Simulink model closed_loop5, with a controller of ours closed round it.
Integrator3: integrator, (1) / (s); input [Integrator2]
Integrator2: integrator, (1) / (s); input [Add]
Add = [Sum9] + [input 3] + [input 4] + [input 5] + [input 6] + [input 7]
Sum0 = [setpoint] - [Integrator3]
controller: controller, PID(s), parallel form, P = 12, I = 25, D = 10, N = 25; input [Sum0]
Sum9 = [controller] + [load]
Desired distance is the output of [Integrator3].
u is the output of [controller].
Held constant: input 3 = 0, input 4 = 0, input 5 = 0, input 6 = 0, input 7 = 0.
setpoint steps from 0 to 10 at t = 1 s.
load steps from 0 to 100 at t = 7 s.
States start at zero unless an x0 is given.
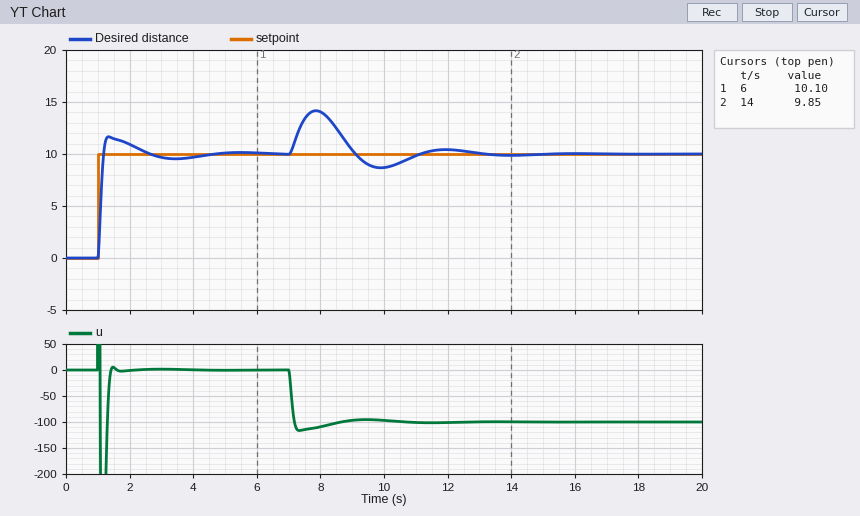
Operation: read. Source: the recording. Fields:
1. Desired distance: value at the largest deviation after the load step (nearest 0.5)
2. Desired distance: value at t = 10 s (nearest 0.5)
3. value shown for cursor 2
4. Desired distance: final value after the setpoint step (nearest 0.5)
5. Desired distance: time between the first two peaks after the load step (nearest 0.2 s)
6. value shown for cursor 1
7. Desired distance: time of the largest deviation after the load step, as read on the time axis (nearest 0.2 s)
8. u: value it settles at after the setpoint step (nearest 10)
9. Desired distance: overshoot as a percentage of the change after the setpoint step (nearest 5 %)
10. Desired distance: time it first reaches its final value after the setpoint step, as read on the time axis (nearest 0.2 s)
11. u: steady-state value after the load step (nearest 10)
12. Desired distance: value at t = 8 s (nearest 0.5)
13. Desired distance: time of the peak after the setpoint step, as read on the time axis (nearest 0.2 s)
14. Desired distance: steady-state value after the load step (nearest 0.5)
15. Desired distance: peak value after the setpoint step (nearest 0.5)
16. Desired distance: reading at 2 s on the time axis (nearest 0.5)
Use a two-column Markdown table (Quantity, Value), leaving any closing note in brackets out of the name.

| Quantity | Value |
|---|---|
| Desired distance: value at the largest deviation after the load step | 14.0 |
| Desired distance: value at t = 10 s | 8.5 |
| value shown for cursor 2 | 9.85 |
| Desired distance: final value after the setpoint step | 10.0 |
| Desired distance: time between the first two peaks after the load step | 4.0 s |
| value shown for cursor 1 | 10.10 |
| Desired distance: time of the largest deviation after the load step, as read on the time axis | 7.8 s |
| u: value it settles at after the setpoint step | 0 |
| Desired distance: overshoot as a percentage of the change after the setpoint step | 15 % |
| Desired distance: time it first reaches its final value after the setpoint step, as read on the time axis | 1.2 s |
| u: steady-state value after the load step | -100 |
| Desired distance: value at t = 8 s | 14.0 |
| Desired distance: time of the peak after the setpoint step, as read on the time axis | 1.4 s |
| Desired distance: steady-state value after the load step | 10.0 |
| Desired distance: peak value after the setpoint step | 11.5 |
| Desired distance: reading at 2 s on the time axis | 11.0 |
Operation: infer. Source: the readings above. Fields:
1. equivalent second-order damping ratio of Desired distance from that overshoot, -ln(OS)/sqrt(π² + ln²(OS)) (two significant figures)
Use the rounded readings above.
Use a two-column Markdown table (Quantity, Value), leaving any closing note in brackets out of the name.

| Quantity | Value |
|---|---|
| equivalent second-order damping ratio of Desired distance from that overshoot, -ln(OS)/sqrt(π² + ln²(OS)) | 0.52 |
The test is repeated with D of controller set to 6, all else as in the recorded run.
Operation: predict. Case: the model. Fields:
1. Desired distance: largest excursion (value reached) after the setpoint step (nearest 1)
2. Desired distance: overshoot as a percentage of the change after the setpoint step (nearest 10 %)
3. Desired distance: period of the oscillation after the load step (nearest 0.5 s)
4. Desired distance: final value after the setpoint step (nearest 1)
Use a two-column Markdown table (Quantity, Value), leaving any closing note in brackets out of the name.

| Quantity | Value |
|---|---|
| Desired distance: largest excursion (value reached) after the setpoint step | 13 |
| Desired distance: overshoot as a percentage of the change after the setpoint step | 30 % |
| Desired distance: period of the oscillation after the load step | 3.0 s |
| Desired distance: final value after the setpoint step | 10 |
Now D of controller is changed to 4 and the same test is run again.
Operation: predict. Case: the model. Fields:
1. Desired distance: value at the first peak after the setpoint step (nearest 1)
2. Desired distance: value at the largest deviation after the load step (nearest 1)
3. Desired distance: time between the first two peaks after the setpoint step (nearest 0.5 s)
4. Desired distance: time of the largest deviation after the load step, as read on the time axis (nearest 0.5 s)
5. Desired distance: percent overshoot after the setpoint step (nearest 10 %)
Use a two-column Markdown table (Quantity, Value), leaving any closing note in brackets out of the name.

| Quantity | Value |
|---|---|
| Desired distance: value at the first peak after the setpoint step | 15 |
| Desired distance: value at the largest deviation after the load step | 17 |
| Desired distance: time between the first two peaks after the setpoint step | 2.0 s |
| Desired distance: time of the largest deviation after the load step, as read on the time axis | 7.5 s |
| Desired distance: percent overshoot after the setpoint step | 50 % |
